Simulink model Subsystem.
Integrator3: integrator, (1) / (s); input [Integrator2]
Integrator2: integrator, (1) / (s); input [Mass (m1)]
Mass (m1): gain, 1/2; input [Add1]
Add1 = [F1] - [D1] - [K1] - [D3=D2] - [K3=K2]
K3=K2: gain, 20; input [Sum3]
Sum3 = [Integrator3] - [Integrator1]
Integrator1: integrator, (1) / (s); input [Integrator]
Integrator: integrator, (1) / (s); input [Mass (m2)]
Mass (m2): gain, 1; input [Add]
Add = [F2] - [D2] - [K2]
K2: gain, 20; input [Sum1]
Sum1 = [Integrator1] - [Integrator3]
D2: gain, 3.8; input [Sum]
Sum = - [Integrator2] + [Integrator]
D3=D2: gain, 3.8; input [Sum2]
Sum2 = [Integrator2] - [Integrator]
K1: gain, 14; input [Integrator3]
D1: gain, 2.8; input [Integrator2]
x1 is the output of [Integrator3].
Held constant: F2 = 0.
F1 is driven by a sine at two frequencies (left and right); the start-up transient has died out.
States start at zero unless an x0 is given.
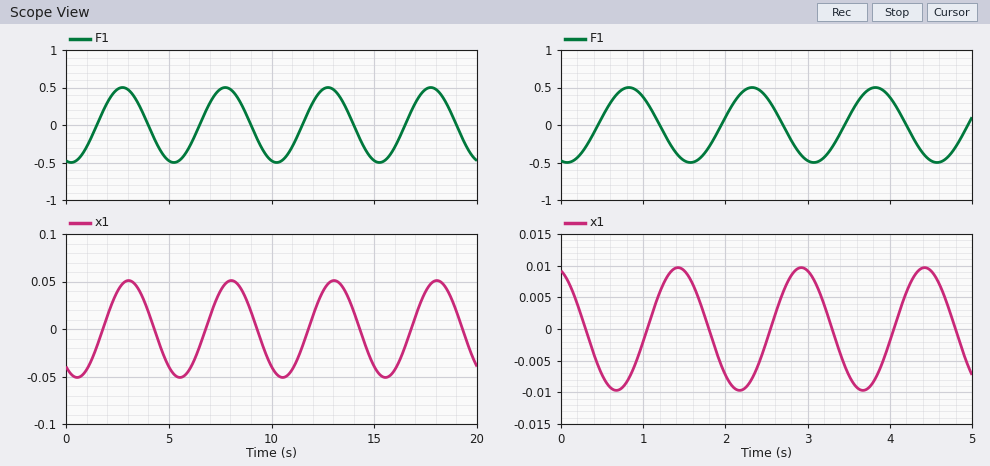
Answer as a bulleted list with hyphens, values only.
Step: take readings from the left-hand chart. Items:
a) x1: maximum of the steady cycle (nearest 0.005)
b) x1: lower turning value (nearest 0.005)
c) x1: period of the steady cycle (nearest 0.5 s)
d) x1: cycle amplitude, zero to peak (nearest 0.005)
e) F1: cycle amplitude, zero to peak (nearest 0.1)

- 0.050
- -0.050
- 5.0 s
- 0.050
- 0.5
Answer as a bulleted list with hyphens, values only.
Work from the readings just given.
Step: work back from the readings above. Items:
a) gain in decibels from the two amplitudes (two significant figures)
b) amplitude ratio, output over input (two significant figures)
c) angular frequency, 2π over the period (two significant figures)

- -20 dB
- 0.10
- 1.3 rad/s
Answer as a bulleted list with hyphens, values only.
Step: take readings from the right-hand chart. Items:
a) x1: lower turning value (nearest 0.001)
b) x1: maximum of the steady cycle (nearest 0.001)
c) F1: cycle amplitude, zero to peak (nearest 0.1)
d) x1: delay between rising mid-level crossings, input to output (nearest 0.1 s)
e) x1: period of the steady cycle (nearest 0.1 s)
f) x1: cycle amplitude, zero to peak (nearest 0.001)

- -0.010
- 0.010
- 0.5
- 0.6 s
- 1.5 s
- 0.010
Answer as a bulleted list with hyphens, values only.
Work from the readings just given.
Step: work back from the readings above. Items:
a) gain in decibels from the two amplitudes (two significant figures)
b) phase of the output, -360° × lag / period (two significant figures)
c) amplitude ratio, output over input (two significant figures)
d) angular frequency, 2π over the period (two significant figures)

- -34 dB
- -140°
- 0.020
- 4.2 rad/s
